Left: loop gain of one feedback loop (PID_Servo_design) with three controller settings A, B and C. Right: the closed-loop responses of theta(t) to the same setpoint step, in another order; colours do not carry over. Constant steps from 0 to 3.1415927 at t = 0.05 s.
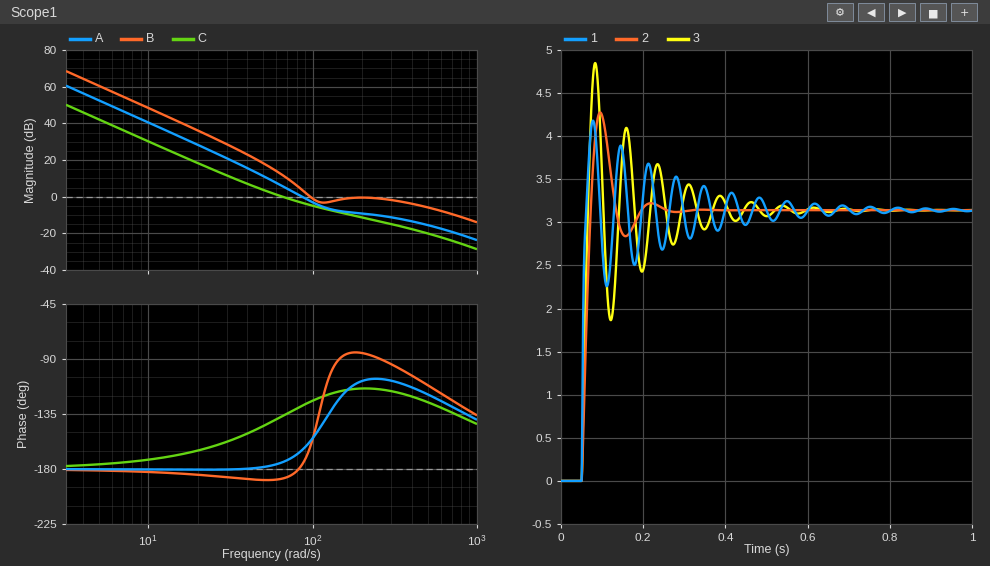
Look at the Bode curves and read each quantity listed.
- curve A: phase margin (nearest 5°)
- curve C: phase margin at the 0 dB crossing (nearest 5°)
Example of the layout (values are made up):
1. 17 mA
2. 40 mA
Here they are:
1. 15°
2. 45°
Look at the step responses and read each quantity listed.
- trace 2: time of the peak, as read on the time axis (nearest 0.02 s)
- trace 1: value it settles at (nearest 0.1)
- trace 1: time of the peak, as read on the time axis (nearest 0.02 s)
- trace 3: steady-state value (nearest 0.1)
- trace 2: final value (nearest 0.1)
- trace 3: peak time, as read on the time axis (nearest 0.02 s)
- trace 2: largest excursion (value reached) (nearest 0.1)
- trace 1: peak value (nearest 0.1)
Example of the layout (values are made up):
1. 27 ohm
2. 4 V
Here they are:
1. 0.10 s
2. 3.1
3. 0.08 s
4. 3.1
5. 3.1
6. 0.08 s
7. 4.3
8. 4.2
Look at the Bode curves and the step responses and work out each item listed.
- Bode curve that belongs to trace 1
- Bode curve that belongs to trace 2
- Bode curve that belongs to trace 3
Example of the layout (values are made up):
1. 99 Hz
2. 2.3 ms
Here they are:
1. B
2. C
3. A
